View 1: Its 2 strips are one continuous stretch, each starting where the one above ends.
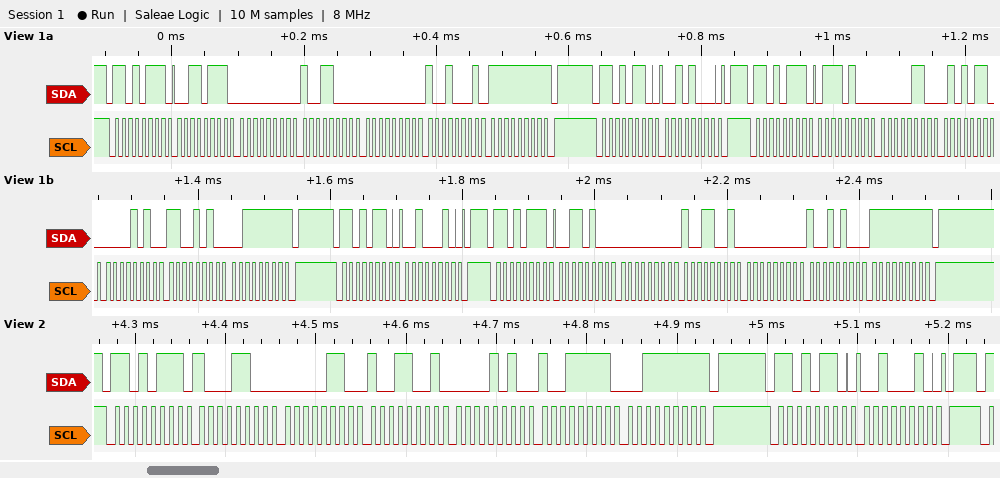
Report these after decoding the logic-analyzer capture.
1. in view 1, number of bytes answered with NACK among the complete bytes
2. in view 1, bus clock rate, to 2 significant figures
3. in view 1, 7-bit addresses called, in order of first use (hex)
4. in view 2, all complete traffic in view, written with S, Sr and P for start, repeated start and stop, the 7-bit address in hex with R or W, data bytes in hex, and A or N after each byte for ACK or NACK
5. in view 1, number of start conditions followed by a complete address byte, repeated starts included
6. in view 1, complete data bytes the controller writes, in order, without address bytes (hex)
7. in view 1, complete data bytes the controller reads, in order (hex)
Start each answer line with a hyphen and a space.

- 3
- 100 kHz
- 0x6B
- S 6BR A 8C A 06 A 99 A 0A A 9F A 3F N P S 6BW A 22 A P
- 5
- 28 22
- 37 00 98 00 91 FF 74 06 56 0A CA 3F 34 00 99 00 94 FF
